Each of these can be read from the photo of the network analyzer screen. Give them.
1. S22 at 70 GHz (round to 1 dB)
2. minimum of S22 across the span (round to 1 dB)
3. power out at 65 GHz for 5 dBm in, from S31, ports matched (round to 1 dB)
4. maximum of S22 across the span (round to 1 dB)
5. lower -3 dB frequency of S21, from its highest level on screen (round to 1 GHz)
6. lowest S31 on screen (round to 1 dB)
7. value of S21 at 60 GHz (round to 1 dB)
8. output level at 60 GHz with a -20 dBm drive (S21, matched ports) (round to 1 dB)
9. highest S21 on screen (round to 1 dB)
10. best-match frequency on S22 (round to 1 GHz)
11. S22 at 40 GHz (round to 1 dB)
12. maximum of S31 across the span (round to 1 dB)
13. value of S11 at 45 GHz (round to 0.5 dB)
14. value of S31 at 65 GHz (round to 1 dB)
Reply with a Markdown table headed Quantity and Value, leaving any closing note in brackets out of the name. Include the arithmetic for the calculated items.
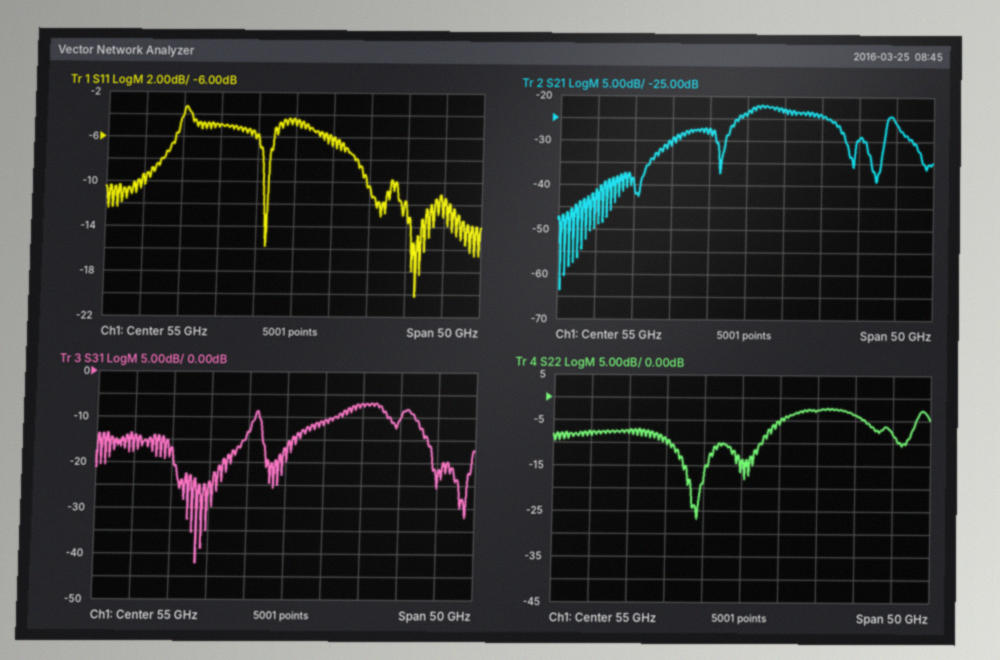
| Quantity | Value |
|---|---|
| S22 at 70 GHz | -4 dB |
| minimum of S22 across the span | -27 dB |
| power out at 65 GHz for 5 dBm in, from S31, ports matched | 5 dBm + (-7 dB) = -2 dBm |
| maximum of S22 across the span | -2 dB |
| lower -3 dB frequency of S21, from its highest level on screen | 54 GHz |
| lowest S31 on screen | -42 dB |
| value of S21 at 60 GHz | -23 dB |
| output level at 60 GHz with a -20 dBm drive (S21, matched ports) | -20 dBm + (-23 dB) = -43 dBm |
| highest S21 on screen | -22 dB |
| best-match frequency on S22 | 49 GHz |
| S22 at 40 GHz | -8 dB |
| maximum of S31 across the span | -7 dB |
| value of S11 at 45 GHz | -5.0 dB |
| value of S31 at 65 GHz | -7 dB |
